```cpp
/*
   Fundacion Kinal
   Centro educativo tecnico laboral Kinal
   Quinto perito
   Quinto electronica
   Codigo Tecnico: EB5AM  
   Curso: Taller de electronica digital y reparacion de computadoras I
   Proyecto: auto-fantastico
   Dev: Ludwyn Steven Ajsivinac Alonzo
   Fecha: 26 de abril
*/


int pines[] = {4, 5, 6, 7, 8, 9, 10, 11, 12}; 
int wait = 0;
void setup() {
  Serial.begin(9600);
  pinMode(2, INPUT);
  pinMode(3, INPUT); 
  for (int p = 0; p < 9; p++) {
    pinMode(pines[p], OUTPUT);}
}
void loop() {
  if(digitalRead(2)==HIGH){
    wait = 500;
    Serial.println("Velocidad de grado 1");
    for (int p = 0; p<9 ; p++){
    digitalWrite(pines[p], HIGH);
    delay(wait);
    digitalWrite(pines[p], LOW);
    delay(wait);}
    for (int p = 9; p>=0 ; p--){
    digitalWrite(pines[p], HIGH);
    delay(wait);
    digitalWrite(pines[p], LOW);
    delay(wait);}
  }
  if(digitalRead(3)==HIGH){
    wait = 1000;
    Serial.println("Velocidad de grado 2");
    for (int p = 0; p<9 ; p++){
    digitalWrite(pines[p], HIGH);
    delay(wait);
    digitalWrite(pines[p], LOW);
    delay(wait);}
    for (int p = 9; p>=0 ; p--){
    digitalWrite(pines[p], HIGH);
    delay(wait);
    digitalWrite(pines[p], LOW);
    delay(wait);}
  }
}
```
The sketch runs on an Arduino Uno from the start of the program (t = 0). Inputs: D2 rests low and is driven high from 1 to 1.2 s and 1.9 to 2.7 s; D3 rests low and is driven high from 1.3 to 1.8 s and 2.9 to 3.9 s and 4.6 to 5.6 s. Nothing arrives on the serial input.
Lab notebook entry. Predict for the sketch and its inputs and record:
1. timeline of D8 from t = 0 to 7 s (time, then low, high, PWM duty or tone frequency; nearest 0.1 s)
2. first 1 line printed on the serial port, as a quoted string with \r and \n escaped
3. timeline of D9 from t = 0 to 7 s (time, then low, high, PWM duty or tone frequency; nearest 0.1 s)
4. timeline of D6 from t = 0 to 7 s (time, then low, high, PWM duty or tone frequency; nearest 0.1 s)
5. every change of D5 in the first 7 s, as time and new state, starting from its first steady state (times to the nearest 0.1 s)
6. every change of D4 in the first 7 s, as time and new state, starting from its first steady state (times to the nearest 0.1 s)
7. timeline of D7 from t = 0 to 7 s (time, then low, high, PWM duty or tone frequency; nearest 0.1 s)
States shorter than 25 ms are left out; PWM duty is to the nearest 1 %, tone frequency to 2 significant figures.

0 s low; 5 s high; 5.5 s low
"Velocidad de grado 1\r\n"
0 s low; 6 s high; 6.5 s low
0 s low; 3 s high; 3.5 s low
0 s low; 2 s high; 2.5 s low
0 s low; 1 s high; 1.5 s low
0 s low; 4 s high; 4.5 s low
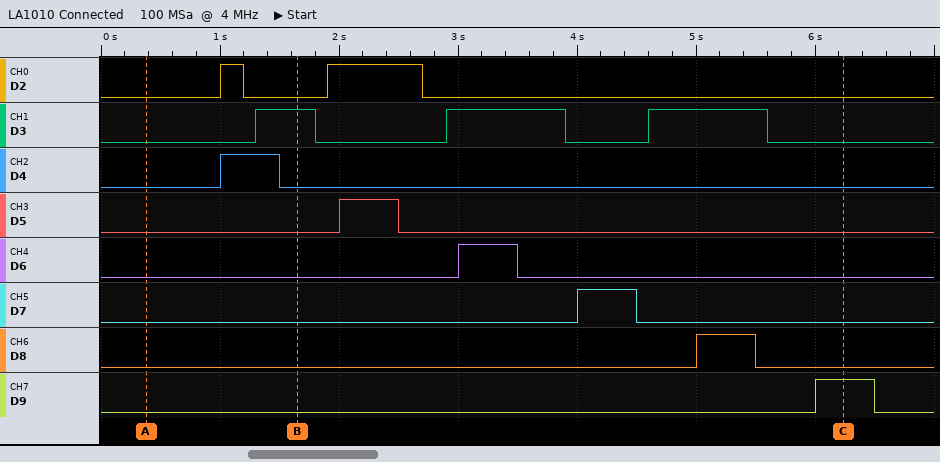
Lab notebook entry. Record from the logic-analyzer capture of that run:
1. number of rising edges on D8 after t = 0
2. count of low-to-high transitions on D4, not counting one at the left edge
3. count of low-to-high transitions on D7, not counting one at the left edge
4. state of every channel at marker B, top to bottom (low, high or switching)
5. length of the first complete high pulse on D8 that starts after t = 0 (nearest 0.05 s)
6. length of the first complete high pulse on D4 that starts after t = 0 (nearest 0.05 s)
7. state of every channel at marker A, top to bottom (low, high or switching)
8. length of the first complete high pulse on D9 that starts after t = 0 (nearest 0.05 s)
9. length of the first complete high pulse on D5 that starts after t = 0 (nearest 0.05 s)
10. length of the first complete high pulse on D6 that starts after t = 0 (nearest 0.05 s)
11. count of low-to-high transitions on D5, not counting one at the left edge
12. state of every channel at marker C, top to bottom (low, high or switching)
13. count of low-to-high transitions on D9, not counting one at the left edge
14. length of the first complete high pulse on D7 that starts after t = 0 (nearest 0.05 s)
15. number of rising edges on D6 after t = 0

1
1
1
D2 low, D3 high, D4 low, D5 low, D6 low, D7 low, D8 low, D9 low
0.50 s
0.50 s
D2 low, D3 low, D4 low, D5 low, D6 low, D7 low, D8 low, D9 low
0.50 s
0.50 s
0.50 s
1
D2 low, D3 low, D4 low, D5 low, D6 low, D7 low, D8 low, D9 high
1
0.50 s
1
